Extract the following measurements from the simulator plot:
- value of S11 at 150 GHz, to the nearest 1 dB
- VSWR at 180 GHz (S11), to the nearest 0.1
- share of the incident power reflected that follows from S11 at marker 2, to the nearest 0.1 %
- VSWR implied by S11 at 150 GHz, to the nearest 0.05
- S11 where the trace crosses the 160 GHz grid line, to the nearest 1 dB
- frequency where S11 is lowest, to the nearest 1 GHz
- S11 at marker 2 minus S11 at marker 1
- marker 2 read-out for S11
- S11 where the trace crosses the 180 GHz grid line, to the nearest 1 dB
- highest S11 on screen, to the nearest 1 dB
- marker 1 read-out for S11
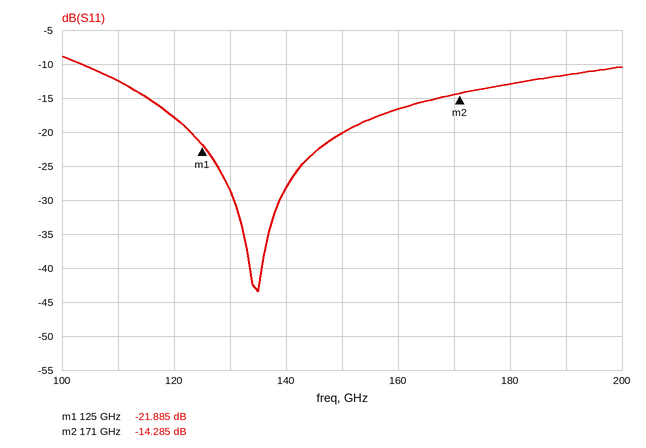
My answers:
-20 dB
1.6
3.7 %
1.20
-17 dB
135 GHz
7.600 dB
-14.285 dB
-13 dB
-9 dB
-21.885 dB
